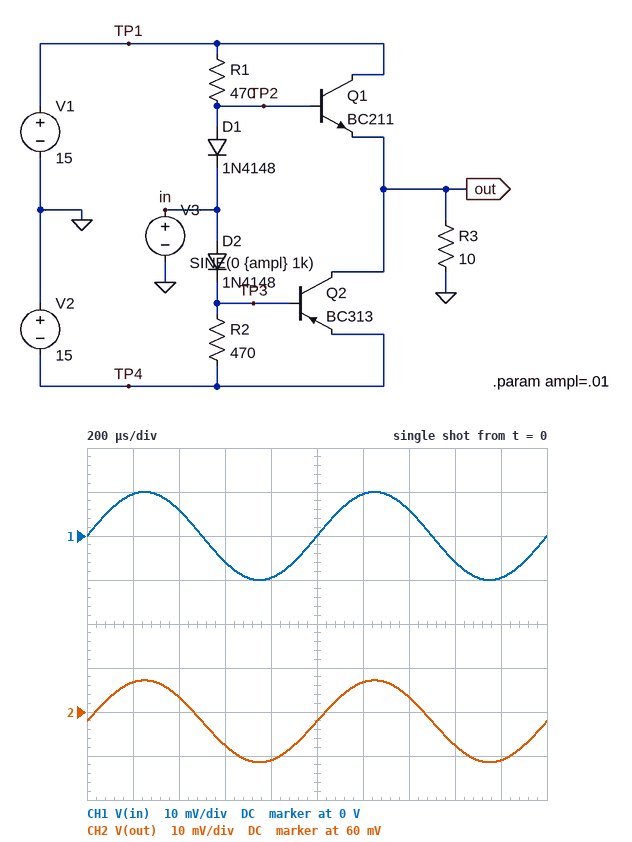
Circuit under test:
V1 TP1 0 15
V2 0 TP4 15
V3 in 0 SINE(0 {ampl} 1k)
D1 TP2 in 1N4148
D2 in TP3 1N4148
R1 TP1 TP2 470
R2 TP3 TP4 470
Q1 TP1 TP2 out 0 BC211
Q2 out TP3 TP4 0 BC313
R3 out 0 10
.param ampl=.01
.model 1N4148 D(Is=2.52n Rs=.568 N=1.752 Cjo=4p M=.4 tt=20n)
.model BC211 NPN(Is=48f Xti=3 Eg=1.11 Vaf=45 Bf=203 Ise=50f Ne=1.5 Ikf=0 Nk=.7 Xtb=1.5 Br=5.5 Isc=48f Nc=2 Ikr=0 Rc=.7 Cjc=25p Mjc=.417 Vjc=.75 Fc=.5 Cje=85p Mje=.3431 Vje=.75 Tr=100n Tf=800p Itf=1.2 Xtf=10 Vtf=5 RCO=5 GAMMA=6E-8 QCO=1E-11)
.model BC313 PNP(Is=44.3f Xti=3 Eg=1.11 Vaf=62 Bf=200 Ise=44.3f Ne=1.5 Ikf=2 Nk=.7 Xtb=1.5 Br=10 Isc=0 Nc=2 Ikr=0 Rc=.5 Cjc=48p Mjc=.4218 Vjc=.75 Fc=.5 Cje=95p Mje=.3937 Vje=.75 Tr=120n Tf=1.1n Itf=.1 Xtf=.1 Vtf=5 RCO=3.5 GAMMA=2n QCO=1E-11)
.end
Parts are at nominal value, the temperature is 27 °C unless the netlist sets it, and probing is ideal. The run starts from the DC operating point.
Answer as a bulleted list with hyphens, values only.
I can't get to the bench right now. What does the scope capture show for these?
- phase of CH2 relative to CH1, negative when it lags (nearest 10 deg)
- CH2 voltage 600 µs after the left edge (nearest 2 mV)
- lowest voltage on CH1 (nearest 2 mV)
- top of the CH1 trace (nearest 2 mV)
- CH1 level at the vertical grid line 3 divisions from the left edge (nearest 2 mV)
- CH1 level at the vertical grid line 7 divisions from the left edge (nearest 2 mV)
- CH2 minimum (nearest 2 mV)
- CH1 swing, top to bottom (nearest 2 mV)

- 0 deg
- 52 mV
- -10 mV
- 10 mV
- -6 mV
- 6 mV
- 48 mV
- 20 mV
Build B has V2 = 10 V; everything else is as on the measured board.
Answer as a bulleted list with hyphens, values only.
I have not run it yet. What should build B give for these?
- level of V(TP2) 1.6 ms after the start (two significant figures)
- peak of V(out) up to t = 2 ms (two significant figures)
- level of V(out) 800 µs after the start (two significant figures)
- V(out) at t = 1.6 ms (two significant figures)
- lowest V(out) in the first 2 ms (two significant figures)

- 750 mV
- 71 mV
- 53 mV
- 56 mV
- 52 mV
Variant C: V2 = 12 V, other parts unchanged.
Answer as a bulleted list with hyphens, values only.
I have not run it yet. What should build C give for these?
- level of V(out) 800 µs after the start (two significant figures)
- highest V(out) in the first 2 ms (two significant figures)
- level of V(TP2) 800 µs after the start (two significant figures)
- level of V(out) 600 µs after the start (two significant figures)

- 51 mV
- 69 mV
- 750 mV
- 54 mV
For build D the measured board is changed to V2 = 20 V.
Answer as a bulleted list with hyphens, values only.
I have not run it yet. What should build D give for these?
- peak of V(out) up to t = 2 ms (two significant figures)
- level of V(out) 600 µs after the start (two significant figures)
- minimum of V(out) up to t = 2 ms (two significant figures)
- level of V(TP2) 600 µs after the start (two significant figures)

- 65 mV
- 50 mV
- 46 mV
- 750 mV
